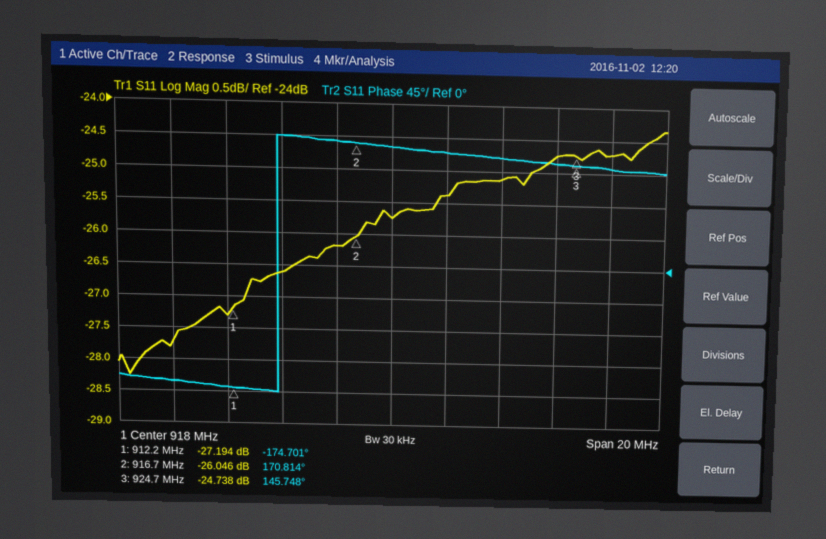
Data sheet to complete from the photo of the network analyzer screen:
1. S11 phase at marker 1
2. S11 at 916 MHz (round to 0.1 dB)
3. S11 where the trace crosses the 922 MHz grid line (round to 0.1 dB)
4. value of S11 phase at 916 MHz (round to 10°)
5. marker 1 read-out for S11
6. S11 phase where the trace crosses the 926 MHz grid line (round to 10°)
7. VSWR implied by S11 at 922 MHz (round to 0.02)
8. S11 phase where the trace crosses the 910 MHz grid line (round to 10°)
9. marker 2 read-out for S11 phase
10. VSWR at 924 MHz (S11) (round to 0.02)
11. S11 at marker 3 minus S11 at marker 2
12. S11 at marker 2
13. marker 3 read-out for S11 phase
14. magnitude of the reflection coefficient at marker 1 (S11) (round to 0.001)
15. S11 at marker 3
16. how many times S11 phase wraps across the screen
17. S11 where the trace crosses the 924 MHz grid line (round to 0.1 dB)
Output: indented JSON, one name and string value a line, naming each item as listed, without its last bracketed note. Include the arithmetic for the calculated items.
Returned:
{
  "S11 phase at marker 1": "-174.701°",
  "S11 at 916 MHz": "-26.2 dB",
  "S11 where the trace crosses the 922 MHz grid line": "-25.1 dB",
  "value of S11 phase at 916 MHz": "170°",
  "marker 1 read-out for S11": "-27.194 dB",
  "S11 phase where the trace crosses the 926 MHz grid line": "140°",
  "VSWR implied by S11 at 922 MHz": "|Γ| = 10^(-25.1/20) = 0.0556; VSWR = (1 + 0.0556)/(1 − 0.0556) ≈ 1.12",
  "S11 phase where the trace crosses the 910 MHz grid line": "-170°",
  "marker 2 read-out for S11 phase": "170.814°",
  "VSWR at 924 MHz (S11)": "|Γ| = 10^(-24.7/20) = 0.0582; VSWR = (1 + 0.0582)/(1 − 0.0582) ≈ 1.12",
  "S11 at marker 3 minus S11 at marker 2": "-24.738 − (-26.046) = 1.308 dB",
  "S11 at marker 2": "-26.046 dB",
  "marker 3 read-out for S11 phase": "145.748°",
  "magnitude of the reflection coefficient at marker 1 (S11)": "10^(-27.194/20) ≈ 0.044",
  "S11 at marker 3": "-24.738 dB",
  "how many times S11 phase wraps across the screen": "1",
  "S11 where the trace crosses the 924 MHz grid line": "-24.7 dB"
}
